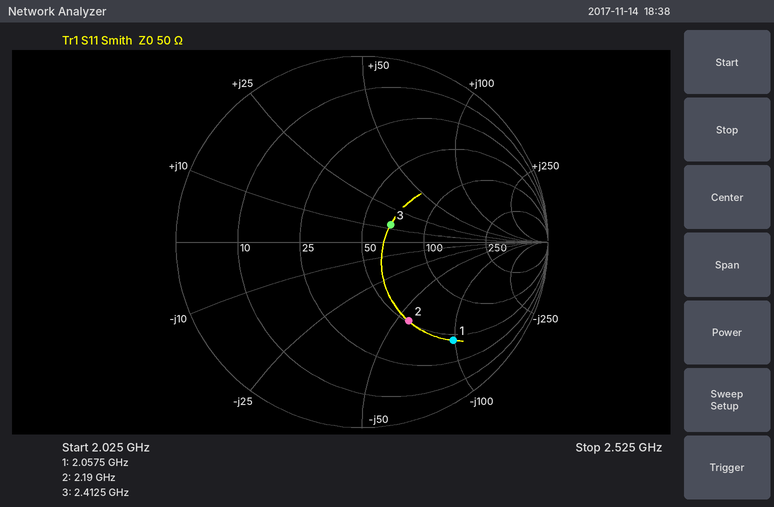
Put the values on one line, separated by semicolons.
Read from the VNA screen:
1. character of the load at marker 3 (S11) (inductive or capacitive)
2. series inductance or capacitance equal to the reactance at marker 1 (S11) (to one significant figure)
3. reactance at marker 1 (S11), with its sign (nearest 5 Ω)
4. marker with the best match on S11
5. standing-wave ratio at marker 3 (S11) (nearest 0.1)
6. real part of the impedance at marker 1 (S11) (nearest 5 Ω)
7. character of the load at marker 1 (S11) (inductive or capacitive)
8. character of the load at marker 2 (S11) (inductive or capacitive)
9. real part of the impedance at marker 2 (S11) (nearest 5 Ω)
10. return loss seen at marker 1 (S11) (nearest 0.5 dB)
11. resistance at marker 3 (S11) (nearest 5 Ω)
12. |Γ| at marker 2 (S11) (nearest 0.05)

inductive; 800 fF; -100 Ω; marker 3; 1.4; 45 Ω; capacitive; capacitive; 50 Ω; 3.0 dB; 65 Ω; 0.50
